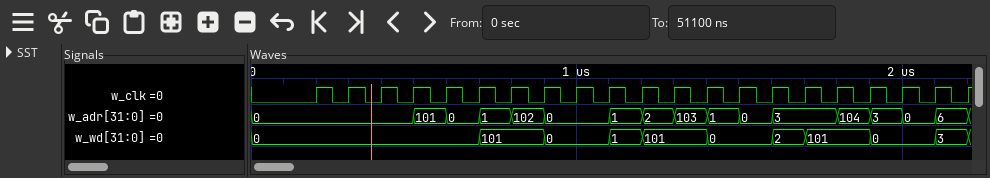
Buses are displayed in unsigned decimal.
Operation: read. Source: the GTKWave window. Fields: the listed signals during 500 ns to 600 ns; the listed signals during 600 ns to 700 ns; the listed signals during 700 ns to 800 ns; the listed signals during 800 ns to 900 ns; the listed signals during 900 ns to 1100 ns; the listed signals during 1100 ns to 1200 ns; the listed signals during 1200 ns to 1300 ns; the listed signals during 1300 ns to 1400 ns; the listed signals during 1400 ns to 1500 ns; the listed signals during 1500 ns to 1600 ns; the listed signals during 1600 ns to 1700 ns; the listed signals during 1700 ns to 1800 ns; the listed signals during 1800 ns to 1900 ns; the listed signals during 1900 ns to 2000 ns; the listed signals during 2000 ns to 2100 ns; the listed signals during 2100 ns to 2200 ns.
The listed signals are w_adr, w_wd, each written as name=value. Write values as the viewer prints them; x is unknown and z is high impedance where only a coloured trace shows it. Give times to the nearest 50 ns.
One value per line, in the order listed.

w_adr=101, w_wd=0
w_adr=0, w_wd=0
w_adr=1, w_wd=101
w_adr=102, w_wd=101
w_adr=0, w_wd=0
w_adr=1, w_wd=1
w_adr=2, w_wd=101
w_adr=103, w_wd=101
w_adr=1, w_wd=0
w_adr=0, w_wd=0
w_adr=3, w_wd=2
w_adr=3, w_wd=101
w_adr=104, w_wd=101
w_adr=3, w_wd=0
w_adr=0, w_wd=0
w_adr=6, w_wd=3
